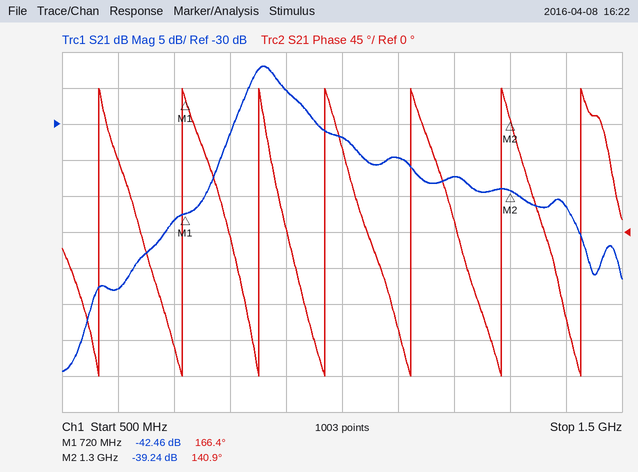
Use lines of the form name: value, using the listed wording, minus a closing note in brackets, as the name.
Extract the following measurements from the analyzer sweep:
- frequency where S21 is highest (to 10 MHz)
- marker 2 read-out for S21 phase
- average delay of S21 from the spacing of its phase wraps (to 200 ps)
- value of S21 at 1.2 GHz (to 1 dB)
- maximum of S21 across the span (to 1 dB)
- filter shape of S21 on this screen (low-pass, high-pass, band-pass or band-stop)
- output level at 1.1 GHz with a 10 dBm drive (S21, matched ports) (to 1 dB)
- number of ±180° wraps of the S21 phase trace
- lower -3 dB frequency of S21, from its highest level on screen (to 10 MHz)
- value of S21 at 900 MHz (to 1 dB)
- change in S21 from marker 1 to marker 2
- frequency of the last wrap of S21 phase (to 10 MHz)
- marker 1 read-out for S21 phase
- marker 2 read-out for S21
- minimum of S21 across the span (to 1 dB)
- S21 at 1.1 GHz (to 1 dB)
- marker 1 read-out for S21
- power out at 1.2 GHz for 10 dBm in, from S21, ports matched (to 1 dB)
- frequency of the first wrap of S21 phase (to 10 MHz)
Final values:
frequency where S21 is highest: 860 MHz
marker 2 read-out for S21 phase: 140.9°
average delay of S21 from the spacing of its phase wraps: 7.0 ns
value of S21 at 1.2 GHz: -37 dB
maximum of S21 across the span: -22 dB
filter shape of S21 on this screen: band-pass
output level at 1.1 GHz with a 10 dBm drive (S21, matched ports): -25 dBm
number of ±180° wraps of the S21 phase trace: 7
lower -3 dB frequency of S21, from its highest level on screen: 830 MHz
value of S21 at 900 MHz: -25 dB
change in S21 from marker 1 to marker 2: 3.22 dB
frequency of the last wrap of S21 phase: 1.43 GHz
marker 1 read-out for S21 phase: 166.4°
marker 2 read-out for S21: -39.24 dB
minimum of S21 across the span: -64 dB
S21 at 1.1 GHz: -35 dB
marker 1 read-out for S21: -42.46 dB
power out at 1.2 GHz for 10 dBm in, from S21, ports matched: -27 dBm
frequency of the first wrap of S21 phase: 570 MHz
